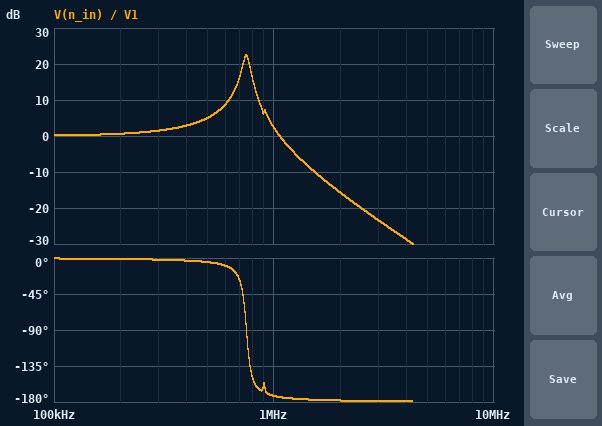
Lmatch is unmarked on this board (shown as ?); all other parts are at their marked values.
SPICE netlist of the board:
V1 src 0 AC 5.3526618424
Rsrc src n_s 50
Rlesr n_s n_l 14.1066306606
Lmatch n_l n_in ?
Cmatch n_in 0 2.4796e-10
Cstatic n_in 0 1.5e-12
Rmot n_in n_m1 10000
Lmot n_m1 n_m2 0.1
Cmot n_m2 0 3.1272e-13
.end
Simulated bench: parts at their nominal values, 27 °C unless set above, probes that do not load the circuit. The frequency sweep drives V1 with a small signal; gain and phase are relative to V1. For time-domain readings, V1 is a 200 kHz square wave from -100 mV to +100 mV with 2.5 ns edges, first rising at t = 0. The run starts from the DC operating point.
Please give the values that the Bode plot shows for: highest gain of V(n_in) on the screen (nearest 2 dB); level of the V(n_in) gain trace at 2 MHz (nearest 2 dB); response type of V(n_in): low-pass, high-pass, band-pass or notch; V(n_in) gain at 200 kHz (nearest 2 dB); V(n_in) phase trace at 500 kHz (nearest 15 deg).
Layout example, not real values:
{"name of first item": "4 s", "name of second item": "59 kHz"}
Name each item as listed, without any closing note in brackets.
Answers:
{"highest gain of V(n_in) on the screen": "22 dB", "level of the V(n_in) gain trace at 2 MHz": "-16 dB", "response type of V(n_in): low-pass, high-pass, band-pass or notch": "low-pass", "V(n_in) gain at 200 kHz": "0 dB", "V(n_in) phase trace at 500 kHz": "0 deg"}
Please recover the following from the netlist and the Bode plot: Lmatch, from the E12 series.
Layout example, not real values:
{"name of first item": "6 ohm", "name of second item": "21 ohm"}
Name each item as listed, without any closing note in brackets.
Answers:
{"Lmatch, from the E12 series": "180 µH"}
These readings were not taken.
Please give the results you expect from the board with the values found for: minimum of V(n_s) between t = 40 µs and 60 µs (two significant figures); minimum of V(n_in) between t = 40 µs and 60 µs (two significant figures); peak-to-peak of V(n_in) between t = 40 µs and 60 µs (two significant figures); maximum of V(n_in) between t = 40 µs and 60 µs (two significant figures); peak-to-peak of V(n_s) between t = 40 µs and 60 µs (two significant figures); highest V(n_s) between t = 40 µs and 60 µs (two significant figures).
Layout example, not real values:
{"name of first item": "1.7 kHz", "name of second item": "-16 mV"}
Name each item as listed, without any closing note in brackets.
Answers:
{"minimum of V(n_s) between t = 40 µs and 60 µs": "-110 mV", "minimum of V(n_in) between t = 40 µs and 60 µs": "-220 mV", "peak-to-peak of V(n_in) between t = 40 µs and 60 µs": "440 mV", "maximum of V(n_in) between t = 40 µs and 60 µs": "220 mV", "peak-to-peak of V(n_s) between t = 40 µs and 60 µs": "210 mV", "highest V(n_s) between t = 40 µs and 60 µs": "110 mV"}
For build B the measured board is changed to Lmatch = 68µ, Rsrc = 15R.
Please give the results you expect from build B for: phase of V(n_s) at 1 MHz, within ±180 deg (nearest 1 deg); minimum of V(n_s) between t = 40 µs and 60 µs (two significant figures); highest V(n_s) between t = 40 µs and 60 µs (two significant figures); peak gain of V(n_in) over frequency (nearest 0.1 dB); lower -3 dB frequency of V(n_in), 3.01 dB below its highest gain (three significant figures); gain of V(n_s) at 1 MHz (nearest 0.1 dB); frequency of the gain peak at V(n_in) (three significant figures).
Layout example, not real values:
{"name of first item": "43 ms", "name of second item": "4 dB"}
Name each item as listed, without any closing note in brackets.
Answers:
{"phase of V(n_s) at 1 MHz, within ±180 deg": "-4 deg", "minimum of V(n_s) between t = 40 µs and 60 µs": "-100 mV", "highest V(n_s) between t = 40 µs and 60 µs": "100 mV", "peak gain of V(n_in) over frequency": "25.1 dB", "lower -3 dB frequency of V(n_in), 3.01 dB below its highest gain": "1.19 MHz", "gain of V(n_s) at 1 MHz": "-0.1 dB", "frequency of the gain peak at V(n_in)": "1.22 MHz"}
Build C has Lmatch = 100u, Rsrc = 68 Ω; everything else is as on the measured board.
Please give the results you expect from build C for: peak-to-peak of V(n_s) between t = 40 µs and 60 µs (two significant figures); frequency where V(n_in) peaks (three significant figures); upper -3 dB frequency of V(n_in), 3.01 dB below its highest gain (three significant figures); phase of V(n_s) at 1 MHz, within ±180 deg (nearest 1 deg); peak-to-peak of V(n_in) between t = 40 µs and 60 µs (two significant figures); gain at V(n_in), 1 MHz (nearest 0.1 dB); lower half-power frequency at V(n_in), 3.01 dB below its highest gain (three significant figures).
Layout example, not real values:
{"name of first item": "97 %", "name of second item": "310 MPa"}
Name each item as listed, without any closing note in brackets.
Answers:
{"peak-to-peak of V(n_s) between t = 40 µs and 60 µs": "250 mV", "frequency where V(n_in) peaks": "1.01 MHz", "upper -3 dB frequency of V(n_in), 3.01 dB below its highest gain": "1.07 MHz", "phase of V(n_s) at 1 MHz, within ±180 deg": "-33 deg", "peak-to-peak of V(n_in) between t = 40 µs and 60 µs": "710 mV", "gain at V(n_in), 1 MHz": "17.7 dB", "lower half-power frequency at V(n_in), 3.01 dB below its highest gain": "942 kHz"}
